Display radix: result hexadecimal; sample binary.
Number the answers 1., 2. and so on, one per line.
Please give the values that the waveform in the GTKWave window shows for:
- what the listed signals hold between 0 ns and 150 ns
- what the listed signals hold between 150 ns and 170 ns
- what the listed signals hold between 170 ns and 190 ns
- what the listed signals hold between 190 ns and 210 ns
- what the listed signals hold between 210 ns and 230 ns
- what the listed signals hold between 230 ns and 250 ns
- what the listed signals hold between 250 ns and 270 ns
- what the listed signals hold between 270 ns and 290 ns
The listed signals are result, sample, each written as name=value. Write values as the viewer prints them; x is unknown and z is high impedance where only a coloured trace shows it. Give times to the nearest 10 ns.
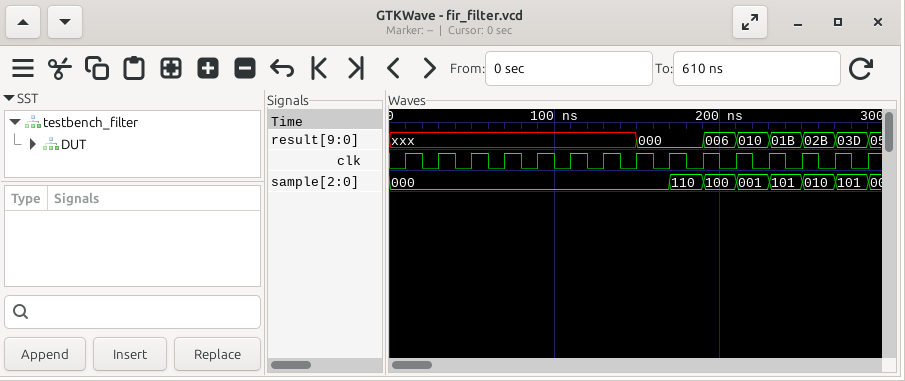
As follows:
1. result=xxx, sample=000
2. result=000, sample=000
3. result=000, sample=110
4. result=006, sample=100
5. result=010, sample=001
6. result=01B, sample=101
7. result=02B, sample=010
8. result=03D, sample=101
